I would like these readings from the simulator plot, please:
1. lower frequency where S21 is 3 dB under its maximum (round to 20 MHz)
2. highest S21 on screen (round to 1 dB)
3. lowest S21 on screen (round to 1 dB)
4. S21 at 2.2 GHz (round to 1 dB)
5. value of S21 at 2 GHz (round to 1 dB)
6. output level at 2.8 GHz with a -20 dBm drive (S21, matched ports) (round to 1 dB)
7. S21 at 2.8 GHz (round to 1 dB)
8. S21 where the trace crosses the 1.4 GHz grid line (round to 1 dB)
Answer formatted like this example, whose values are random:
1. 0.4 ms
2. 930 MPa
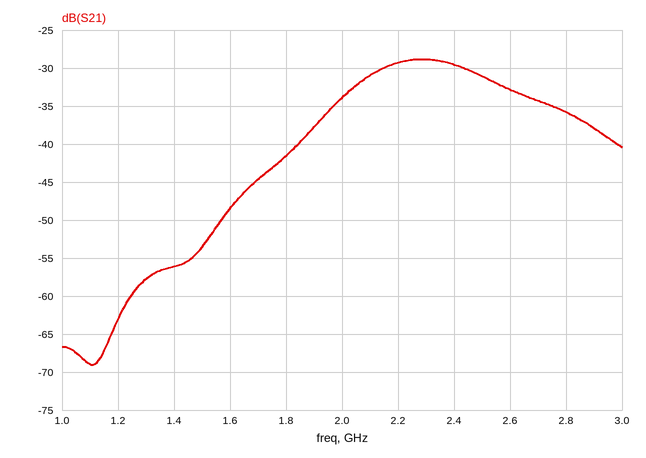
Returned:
1. 2.06 GHz
2. -29 dB
3. -69 dB
4. -29 dB
5. -34 dB
6. -56 dBm
7. -36 dB
8. -56 dB
